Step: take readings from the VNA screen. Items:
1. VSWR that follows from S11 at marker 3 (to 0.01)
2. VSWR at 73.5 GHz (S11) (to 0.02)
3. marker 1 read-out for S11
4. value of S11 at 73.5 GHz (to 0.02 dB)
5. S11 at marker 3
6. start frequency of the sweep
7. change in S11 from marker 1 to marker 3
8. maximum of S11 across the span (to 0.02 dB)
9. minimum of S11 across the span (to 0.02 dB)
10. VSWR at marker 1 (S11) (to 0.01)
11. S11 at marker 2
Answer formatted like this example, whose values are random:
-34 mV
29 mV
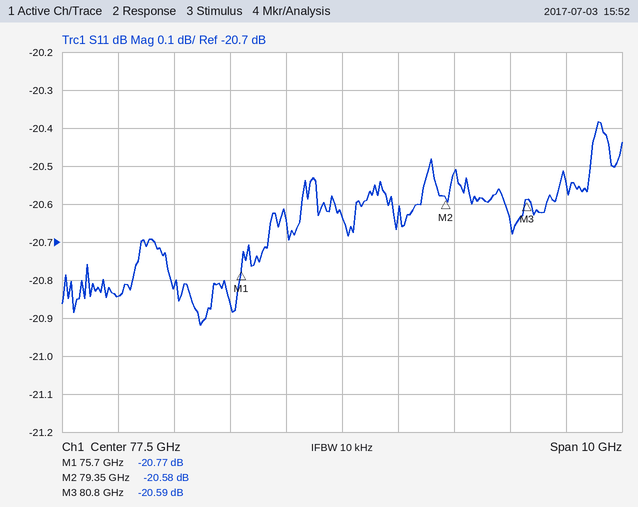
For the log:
1.21
1.20
-20.77 dB
-20.84 dB
-20.59 dB
72.5 GHz
0.18 dB
-20.38 dB
-20.92 dB
1.20
-20.58 dB
